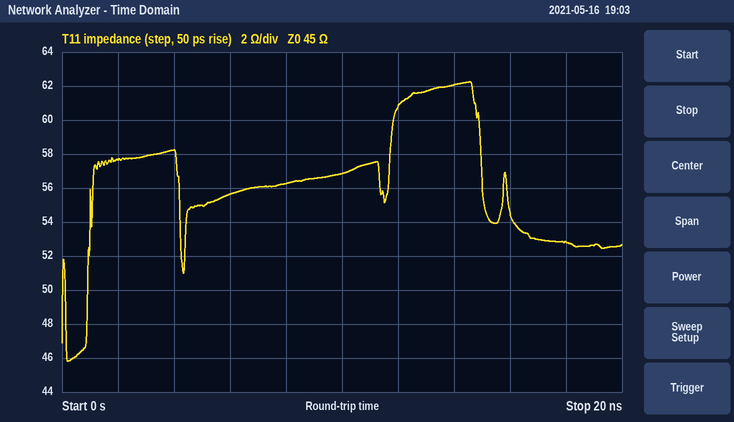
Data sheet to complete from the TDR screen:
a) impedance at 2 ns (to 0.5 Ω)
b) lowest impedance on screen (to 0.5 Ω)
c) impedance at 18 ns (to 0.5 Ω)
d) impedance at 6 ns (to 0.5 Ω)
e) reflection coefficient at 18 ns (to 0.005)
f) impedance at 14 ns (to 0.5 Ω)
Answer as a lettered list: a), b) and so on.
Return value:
a) 57.5 Ω
b) 46.0 Ω
c) 53.0 Ω
d) 55.5 Ω
e) +0.080
f) 62.0 Ω
